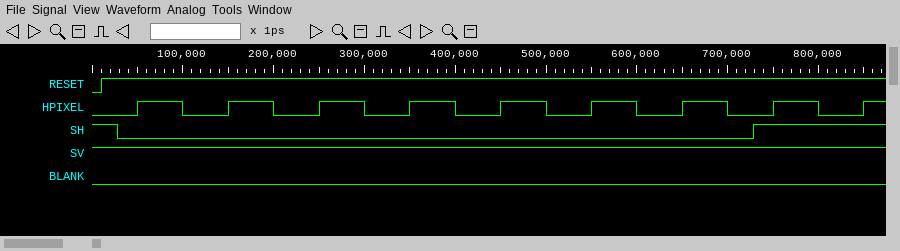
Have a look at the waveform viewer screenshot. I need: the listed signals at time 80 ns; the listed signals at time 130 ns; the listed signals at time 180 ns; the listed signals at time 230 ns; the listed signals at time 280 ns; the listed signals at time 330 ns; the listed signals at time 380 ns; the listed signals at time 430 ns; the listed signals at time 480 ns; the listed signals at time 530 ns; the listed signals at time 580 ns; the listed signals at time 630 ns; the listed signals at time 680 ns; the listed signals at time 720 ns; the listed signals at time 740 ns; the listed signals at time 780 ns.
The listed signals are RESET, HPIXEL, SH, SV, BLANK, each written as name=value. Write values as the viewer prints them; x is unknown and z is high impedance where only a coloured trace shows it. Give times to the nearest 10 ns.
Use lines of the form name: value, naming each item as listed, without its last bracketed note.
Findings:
the listed signals at time 80 ns: RESET=1, HPIXEL=1, SH=0, SV=1, BLANK=0
the listed signals at time 130 ns: RESET=1, HPIXEL=0, SH=0, SV=1, BLANK=0
the listed signals at time 180 ns: RESET=1, HPIXEL=1, SH=0, SV=1, BLANK=0
the listed signals at time 230 ns: RESET=1, HPIXEL=0, SH=0, SV=1, BLANK=0
the listed signals at time 280 ns: RESET=1, HPIXEL=1, SH=0, SV=1, BLANK=0
the listed signals at time 330 ns: RESET=1, HPIXEL=0, SH=0, SV=1, BLANK=0
the listed signals at time 380 ns: RESET=1, HPIXEL=1, SH=0, SV=1, BLANK=0
the listed signals at time 430 ns: RESET=1, HPIXEL=0, SH=0, SV=1, BLANK=0
the listed signals at time 480 ns: RESET=1, HPIXEL=1, SH=0, SV=1, BLANK=0
the listed signals at time 530 ns: RESET=1, HPIXEL=0, SH=0, SV=1, BLANK=0
the listed signals at time 580 ns: RESET=1, HPIXEL=1, SH=0, SV=1, BLANK=0
the listed signals at time 630 ns: RESET=1, HPIXEL=0, SH=0, SV=1, BLANK=0
the listed signals at time 680 ns: RESET=1, HPIXEL=1, SH=0, SV=1, BLANK=0
the listed signals at time 720 ns: RESET=1, HPIXEL=0, SH=0, SV=1, BLANK=0
the listed signals at time 740 ns: RESET=1, HPIXEL=0, SH=1, SV=1, BLANK=0
the listed signals at time 780 ns: RESET=1, HPIXEL=1, SH=1, SV=1, BLANK=0
